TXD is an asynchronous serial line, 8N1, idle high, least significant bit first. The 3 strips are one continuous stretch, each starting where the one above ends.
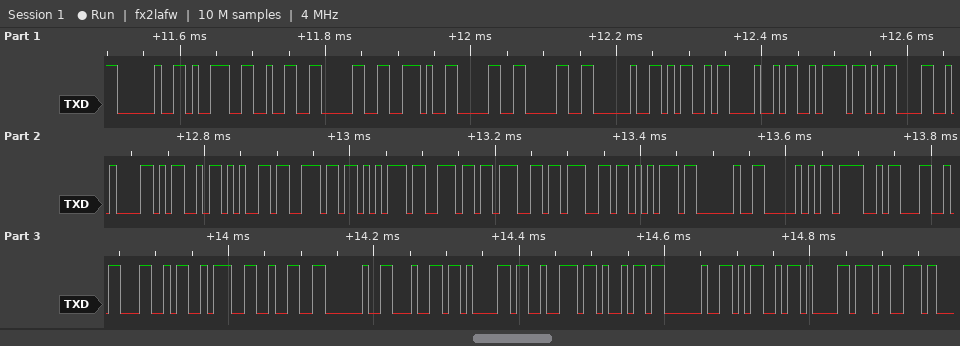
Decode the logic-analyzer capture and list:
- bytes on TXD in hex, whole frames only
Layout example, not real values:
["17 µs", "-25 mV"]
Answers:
["20 39 32 30 2E 30 30 20 4D 48 7A 0D 0A 4D 65 6E 75 6E 67 67 75 20 50 4F 4C 4C 3A 32 20 64 61 72 69 20 4D 61 73"]
